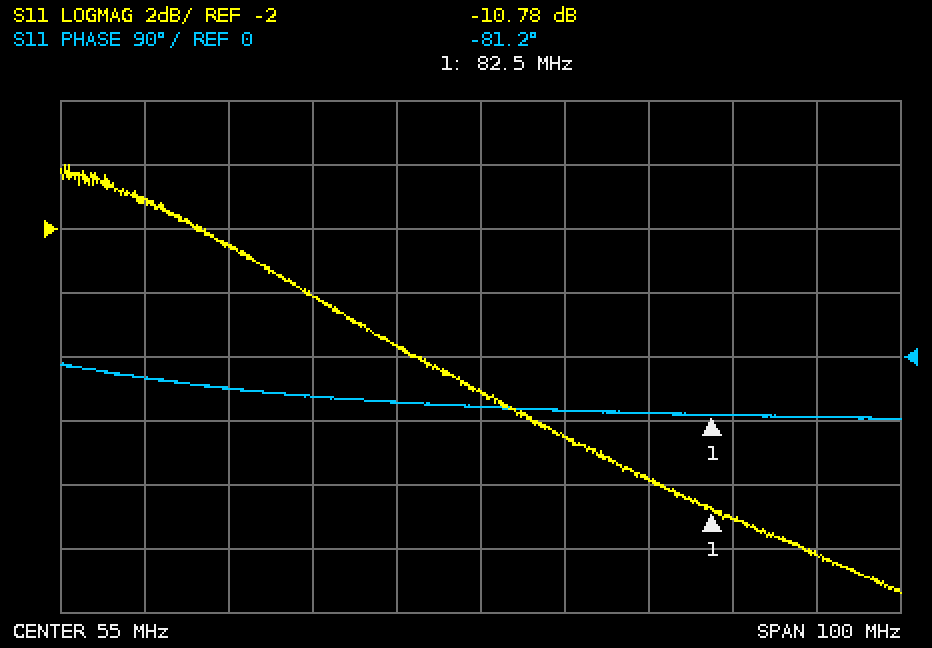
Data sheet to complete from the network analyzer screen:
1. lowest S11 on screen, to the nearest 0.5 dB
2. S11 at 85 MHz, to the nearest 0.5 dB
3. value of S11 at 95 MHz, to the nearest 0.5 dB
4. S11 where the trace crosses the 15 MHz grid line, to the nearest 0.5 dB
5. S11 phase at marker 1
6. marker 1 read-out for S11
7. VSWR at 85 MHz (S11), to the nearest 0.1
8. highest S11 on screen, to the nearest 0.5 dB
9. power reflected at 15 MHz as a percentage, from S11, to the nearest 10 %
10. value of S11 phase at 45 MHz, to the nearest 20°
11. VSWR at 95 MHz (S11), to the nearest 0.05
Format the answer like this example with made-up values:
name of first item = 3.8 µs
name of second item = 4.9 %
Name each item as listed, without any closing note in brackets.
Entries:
lowest S11 on screen, to the nearest 0.5 dB = -13.5 dB
S11 at 85 MHz, to the nearest 0.5 dB = -11.0 dB
value of S11 at 95 MHz, to the nearest 0.5 dB = -12.0 dB
S11 where the trace crosses the 15 MHz grid line, to the nearest 0.5 dB = -1.0 dB
S11 phase at marker 1 = -81.2°
marker 1 read-out for S11 = -10.78 dB
VSWR at 85 MHz (S11), to the nearest 0.1 = 1.8
highest S11 on screen, to the nearest 0.5 dB = 0.0 dB
power reflected at 15 MHz as a percentage, from S11, to the nearest 10 % = 80 %
value of S11 phase at 45 MHz, to the nearest 20° = -60°
VSWR at 95 MHz (S11), to the nearest 0.05 = 1.65
